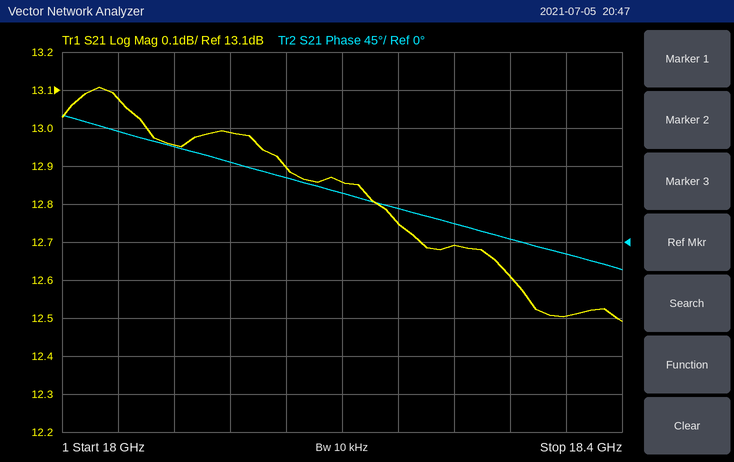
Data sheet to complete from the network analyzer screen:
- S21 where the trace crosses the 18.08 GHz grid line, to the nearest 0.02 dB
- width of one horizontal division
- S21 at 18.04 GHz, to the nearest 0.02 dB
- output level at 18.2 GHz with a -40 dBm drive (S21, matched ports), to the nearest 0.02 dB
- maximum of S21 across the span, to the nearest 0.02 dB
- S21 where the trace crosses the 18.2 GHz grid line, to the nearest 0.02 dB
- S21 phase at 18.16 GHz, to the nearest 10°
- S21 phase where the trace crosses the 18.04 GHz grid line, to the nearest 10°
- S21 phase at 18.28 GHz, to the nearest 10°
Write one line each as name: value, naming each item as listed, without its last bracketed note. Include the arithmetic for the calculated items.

S21 where the trace crosses the 18.08 GHz grid line, to the nearest 0.02 dB: 12.96 dB
width of one horizontal division: 40 MHz
S21 at 18.04 GHz, to the nearest 0.02 dB: 13.08 dB
output level at 18.2 GHz with a -40 dBm drive (S21, matched ports), to the nearest 0.02 dB: -40 dBm + (12.86 dB) = -27.14 dBm
maximum of S21 across the span, to the nearest 0.02 dB: 13.10 dB
S21 where the trace crosses the 18.2 GHz grid line, to the nearest 0.02 dB: 12.86 dB
S21 phase at 18.16 GHz, to the nearest 10°: 80°
S21 phase where the trace crosses the 18.04 GHz grid line, to the nearest 10°: 130°
S21 phase at 18.28 GHz, to the nearest 10°: 20°
